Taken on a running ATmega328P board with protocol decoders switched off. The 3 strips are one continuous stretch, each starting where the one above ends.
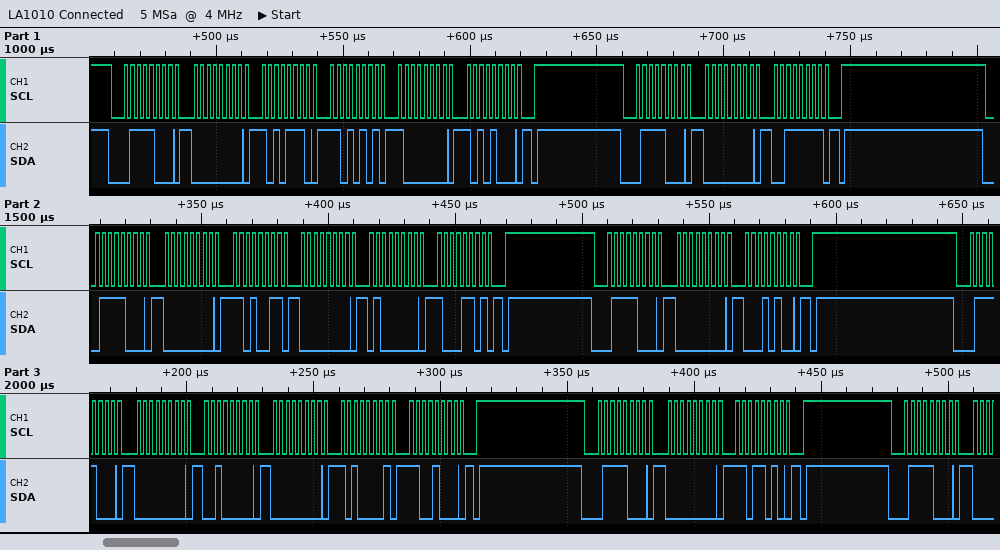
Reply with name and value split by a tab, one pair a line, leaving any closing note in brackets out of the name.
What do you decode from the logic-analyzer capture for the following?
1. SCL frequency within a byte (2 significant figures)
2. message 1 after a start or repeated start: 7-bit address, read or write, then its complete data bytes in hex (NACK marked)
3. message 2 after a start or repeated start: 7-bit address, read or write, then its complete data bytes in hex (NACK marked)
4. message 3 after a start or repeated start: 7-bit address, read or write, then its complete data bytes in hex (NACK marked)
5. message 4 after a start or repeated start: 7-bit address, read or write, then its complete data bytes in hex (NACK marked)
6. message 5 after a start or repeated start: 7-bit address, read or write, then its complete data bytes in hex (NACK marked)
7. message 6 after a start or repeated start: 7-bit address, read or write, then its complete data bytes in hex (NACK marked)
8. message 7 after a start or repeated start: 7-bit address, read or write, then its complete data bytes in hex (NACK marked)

SCL frequency within a byte	400 kHz
message 1 after a start or repeated start: 7-bit address, read or write, then its complete data bytes in hex	0x3C write: 00 AE D5 80 A8
message 2 after a start or repeated start: 7-bit address, read or write, then its complete data bytes in hex	0x3C write: 00 3F
message 3 after a start or repeated start: 7-bit address, read or write, then its complete data bytes in hex	0x3C write: 00 D3 00 40 8D
message 4 after a start or repeated start: 7-bit address, read or write, then its complete data bytes in hex	0x3C write: 00 14
message 5 after a start or repeated start: 7-bit address, read or write, then its complete data bytes in hex	0x3C write: 00 20 00 A1 C8
message 6 after a start or repeated start: 7-bit address, read or write, then its complete data bytes in hex	0x3C write: 00 DA
message 7 after a start or repeated start: 7-bit address, read or write, then its complete data bytes in hex	0x3C write
